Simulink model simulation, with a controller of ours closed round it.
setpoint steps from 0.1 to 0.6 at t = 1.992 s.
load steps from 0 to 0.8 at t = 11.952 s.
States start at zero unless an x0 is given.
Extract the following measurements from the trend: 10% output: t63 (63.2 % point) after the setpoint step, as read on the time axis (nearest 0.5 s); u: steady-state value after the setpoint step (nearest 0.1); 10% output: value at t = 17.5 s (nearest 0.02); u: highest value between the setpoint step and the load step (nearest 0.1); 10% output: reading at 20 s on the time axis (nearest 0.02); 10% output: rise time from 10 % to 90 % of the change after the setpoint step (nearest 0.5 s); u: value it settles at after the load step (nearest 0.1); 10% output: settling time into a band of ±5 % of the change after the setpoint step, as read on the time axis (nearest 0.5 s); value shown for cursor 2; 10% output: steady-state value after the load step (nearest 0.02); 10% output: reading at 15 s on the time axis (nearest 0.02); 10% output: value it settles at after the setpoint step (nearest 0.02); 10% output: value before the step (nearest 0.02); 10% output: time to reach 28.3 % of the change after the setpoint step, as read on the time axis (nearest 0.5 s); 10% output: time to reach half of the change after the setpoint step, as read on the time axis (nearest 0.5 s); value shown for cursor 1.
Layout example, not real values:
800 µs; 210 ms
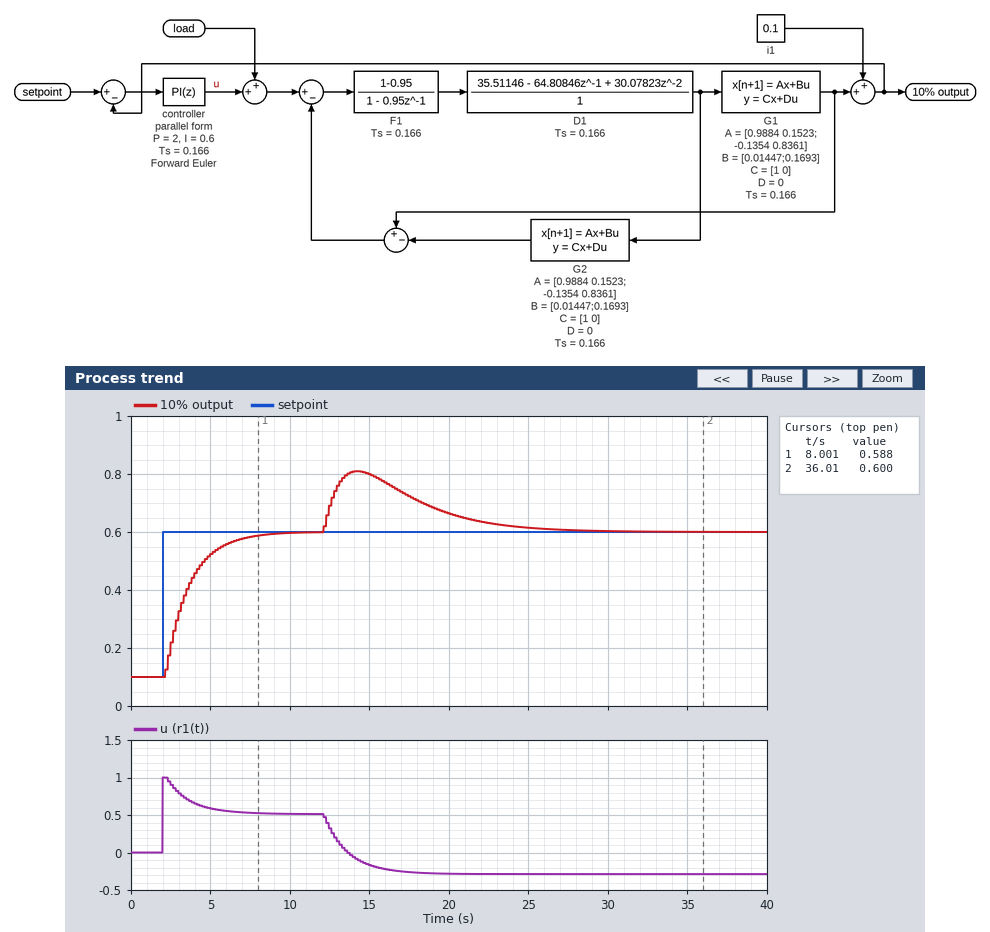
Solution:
3.5 s; 0.5; 0.72; 1.0; 0.66; 3.5 s; -0.3; 7.0 s; 0.600; 0.60; 0.80; 0.60; 0.10; 2.5 s; 3.0 s; 0.588
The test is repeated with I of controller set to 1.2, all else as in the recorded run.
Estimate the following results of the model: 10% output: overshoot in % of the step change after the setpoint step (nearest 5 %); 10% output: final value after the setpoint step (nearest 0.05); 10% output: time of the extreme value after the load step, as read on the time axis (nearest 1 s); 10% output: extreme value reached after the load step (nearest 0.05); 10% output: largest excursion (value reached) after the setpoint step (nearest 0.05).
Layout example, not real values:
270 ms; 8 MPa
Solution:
10 %; 0.60; 14 s; 0.80; 0.65
